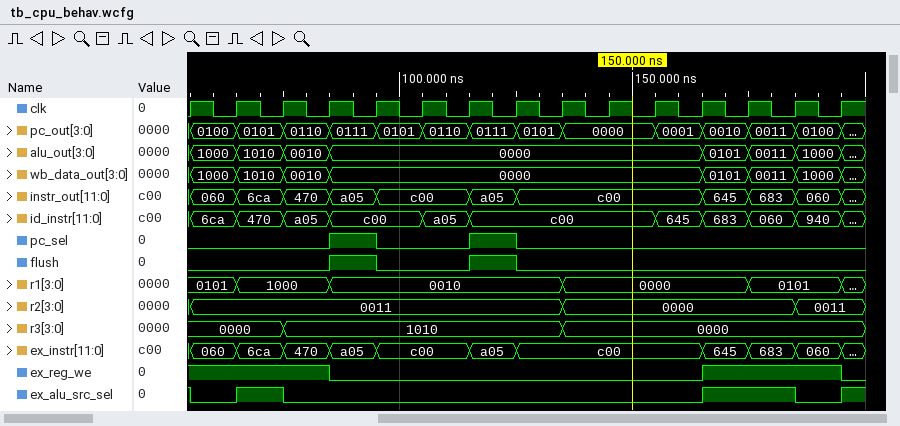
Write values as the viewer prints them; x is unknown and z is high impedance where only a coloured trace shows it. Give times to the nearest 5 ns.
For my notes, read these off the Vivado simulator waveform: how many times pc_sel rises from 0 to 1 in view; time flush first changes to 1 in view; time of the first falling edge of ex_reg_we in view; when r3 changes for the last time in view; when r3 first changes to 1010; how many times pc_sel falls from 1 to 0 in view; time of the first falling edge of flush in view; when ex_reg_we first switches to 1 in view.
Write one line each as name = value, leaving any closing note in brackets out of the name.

how many times pc_sel rises from 0 to 1 in view = 2
time flush first changes to 1 in view = 85 ns
time of the first falling edge of ex_reg_we in view = 85 ns
when r3 changes for the last time in view = 135 ns
when r3 first changes to 1010 = 75 ns
how many times pc_sel falls from 1 to 0 in view = 2
time of the first falling edge of flush in view = 95 ns
when ex_reg_we first switches to 1 in view = 165 ns
